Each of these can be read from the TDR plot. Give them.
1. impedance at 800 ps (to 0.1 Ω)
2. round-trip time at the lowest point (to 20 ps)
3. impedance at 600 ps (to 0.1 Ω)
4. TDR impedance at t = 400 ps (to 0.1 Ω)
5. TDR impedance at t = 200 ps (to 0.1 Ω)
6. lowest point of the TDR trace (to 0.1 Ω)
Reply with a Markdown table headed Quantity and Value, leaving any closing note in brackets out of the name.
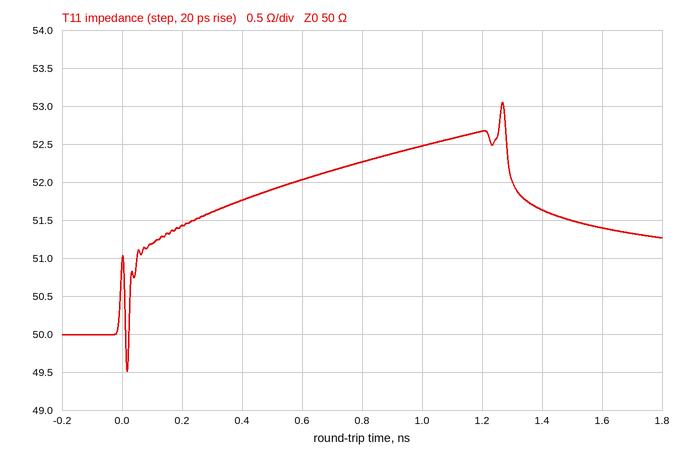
| Quantity | Value |
|---|---|
| impedance at 800 ps | 52.3 Ω |
| round-trip time at the lowest point | 20 ps |
| impedance at 600 ps | 52.0 Ω |
| TDR impedance at t = 400 ps | 51.8 Ω |
| TDR impedance at t = 200 ps | 51.4 Ω |
| lowest point of the TDR trace | 49.5 Ω |
